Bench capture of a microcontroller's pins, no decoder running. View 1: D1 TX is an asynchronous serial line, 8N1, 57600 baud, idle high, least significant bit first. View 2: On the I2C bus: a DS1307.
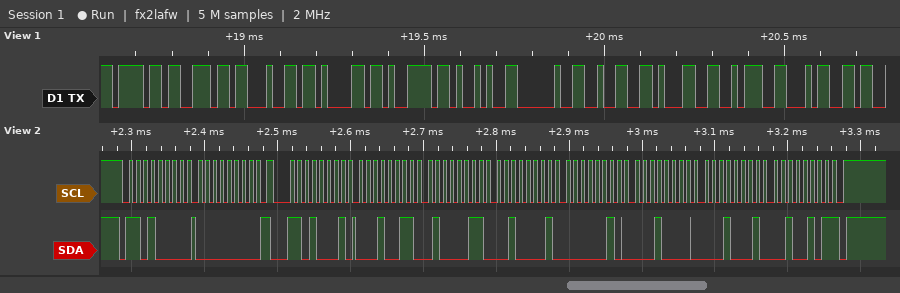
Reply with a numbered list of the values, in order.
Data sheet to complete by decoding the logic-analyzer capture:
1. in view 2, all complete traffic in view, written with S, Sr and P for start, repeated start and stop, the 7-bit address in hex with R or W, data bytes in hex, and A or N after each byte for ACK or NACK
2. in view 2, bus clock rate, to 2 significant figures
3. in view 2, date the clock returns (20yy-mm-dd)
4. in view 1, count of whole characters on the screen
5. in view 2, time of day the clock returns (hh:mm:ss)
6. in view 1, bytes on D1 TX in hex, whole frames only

1. S 68W A 00 A Sr 68R A 13 A 43 A 21 A 02 A 10 A 11 A 25 N P
2. 100 kHz
3. 2025-11-10
4. 11
5. 21:43:13
6. 6F 6E 64 61 79 29 20 32 31 3A 34
